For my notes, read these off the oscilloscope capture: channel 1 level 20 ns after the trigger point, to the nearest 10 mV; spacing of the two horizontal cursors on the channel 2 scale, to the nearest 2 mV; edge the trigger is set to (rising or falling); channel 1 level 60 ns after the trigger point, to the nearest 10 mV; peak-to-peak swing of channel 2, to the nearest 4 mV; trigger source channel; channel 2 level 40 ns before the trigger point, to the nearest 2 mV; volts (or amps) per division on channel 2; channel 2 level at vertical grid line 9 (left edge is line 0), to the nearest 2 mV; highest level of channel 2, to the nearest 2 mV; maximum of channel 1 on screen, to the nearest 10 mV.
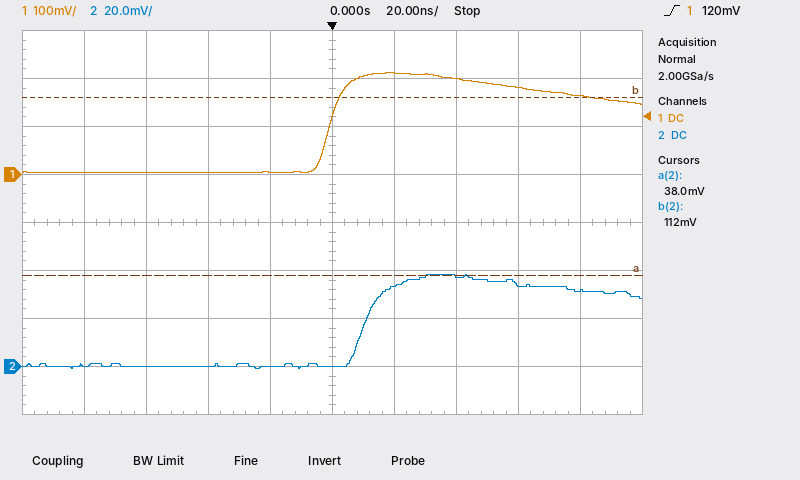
210 mV
74 mV
rising
180 mV
40 mV
channel 1
0 mV
20 mV
32 mV
38 mV
210 mV
